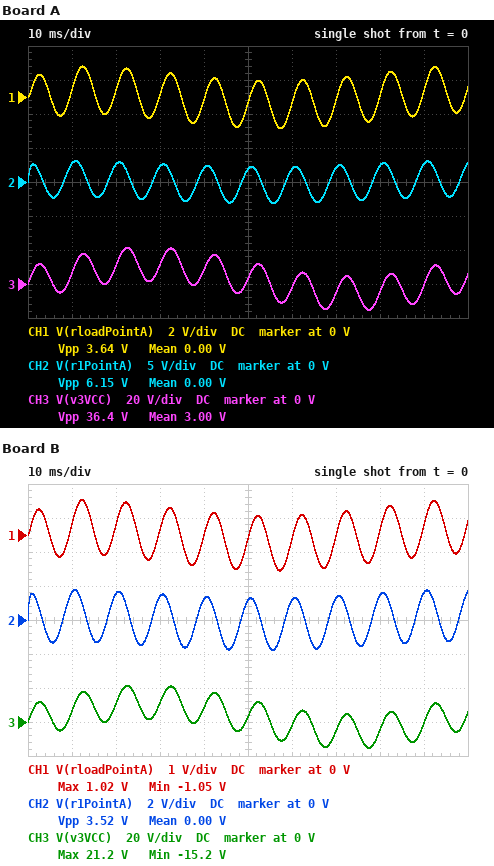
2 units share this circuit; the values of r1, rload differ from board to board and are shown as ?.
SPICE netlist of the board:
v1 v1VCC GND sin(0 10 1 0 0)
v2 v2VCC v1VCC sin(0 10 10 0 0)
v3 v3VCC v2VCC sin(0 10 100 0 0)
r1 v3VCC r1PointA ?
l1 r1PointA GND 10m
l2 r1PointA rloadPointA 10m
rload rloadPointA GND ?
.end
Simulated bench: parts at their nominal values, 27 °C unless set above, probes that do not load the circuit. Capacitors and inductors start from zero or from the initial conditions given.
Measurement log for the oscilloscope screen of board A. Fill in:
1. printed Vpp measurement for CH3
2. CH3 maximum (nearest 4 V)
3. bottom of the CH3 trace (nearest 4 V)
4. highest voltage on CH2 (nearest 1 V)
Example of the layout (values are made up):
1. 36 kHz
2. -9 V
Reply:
1. 36.4 V
2. 20 V
3. -16 V
4. 3 V
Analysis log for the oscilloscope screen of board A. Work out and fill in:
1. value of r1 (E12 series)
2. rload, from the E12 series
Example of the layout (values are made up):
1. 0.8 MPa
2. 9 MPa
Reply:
1. 12 Ω
2. 3.9 Ω
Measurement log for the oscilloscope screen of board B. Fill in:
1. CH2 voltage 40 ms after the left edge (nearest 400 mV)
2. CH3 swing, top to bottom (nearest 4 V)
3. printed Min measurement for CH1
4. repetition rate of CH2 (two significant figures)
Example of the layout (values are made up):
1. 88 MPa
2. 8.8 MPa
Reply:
1. 1.2 V
2. 36 V
3. -1.05 V
4. 100 Hz
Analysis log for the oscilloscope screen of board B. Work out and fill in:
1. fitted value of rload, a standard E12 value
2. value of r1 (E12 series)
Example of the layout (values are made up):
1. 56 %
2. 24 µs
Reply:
1. 3.9 Ω
2. 22 Ω
